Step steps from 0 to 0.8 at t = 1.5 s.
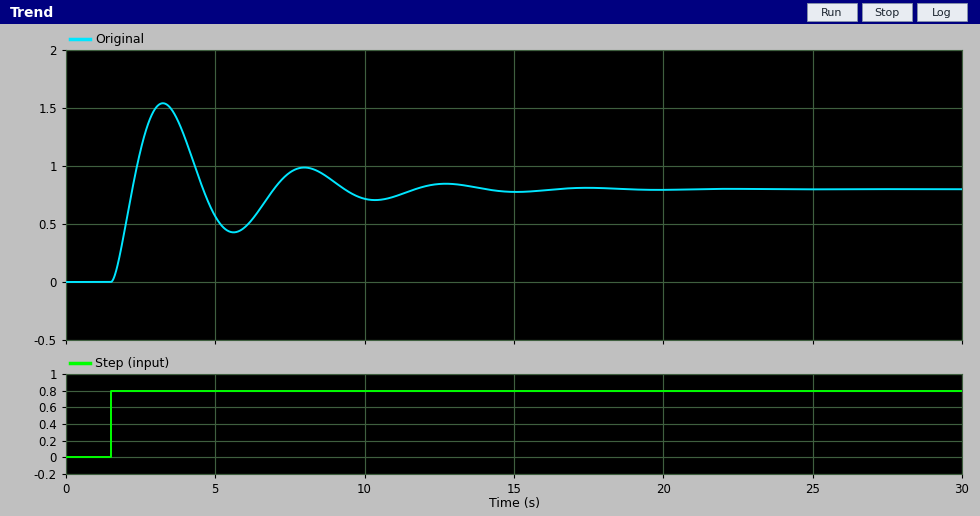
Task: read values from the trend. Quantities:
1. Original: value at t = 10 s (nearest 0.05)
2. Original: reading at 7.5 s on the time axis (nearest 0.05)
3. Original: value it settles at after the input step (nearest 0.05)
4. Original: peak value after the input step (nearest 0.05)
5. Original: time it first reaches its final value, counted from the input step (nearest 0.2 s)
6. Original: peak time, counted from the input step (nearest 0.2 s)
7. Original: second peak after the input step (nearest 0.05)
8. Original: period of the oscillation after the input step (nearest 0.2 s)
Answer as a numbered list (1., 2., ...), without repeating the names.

1. 0.70
2. 0.95
3. 0.80
4. 1.55
5. 0.8 s
6. 1.8 s
7. 1.00
8. 4.8 s
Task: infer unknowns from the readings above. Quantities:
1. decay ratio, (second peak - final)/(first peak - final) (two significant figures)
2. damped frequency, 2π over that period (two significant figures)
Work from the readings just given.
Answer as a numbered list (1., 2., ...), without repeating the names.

1. 0.27
2. 1.3 rad/s
